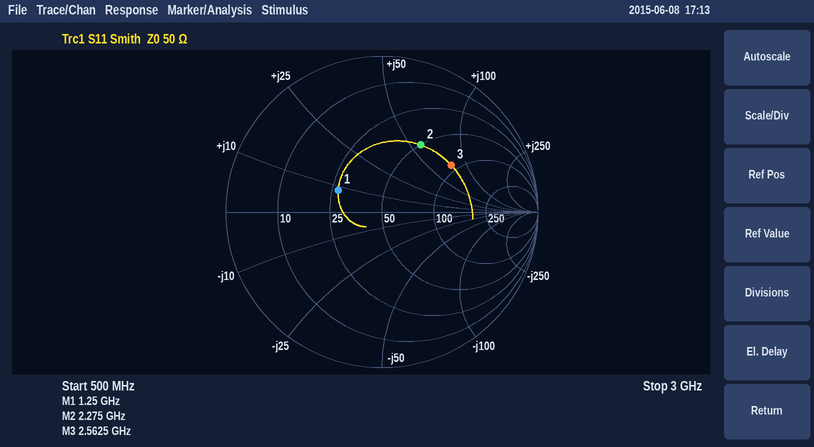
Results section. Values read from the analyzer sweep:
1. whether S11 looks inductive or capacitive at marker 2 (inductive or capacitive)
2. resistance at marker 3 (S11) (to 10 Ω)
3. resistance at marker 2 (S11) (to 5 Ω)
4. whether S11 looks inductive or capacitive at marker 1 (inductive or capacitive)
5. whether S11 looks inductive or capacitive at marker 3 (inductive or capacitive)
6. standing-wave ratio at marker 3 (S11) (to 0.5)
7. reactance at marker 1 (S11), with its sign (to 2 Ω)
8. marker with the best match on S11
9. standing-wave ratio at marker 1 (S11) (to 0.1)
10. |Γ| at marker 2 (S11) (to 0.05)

inductive
90 Ω
50 Ω
inductive
inductive
3.5
+8 Ω
marker 1
1.9
0.50
